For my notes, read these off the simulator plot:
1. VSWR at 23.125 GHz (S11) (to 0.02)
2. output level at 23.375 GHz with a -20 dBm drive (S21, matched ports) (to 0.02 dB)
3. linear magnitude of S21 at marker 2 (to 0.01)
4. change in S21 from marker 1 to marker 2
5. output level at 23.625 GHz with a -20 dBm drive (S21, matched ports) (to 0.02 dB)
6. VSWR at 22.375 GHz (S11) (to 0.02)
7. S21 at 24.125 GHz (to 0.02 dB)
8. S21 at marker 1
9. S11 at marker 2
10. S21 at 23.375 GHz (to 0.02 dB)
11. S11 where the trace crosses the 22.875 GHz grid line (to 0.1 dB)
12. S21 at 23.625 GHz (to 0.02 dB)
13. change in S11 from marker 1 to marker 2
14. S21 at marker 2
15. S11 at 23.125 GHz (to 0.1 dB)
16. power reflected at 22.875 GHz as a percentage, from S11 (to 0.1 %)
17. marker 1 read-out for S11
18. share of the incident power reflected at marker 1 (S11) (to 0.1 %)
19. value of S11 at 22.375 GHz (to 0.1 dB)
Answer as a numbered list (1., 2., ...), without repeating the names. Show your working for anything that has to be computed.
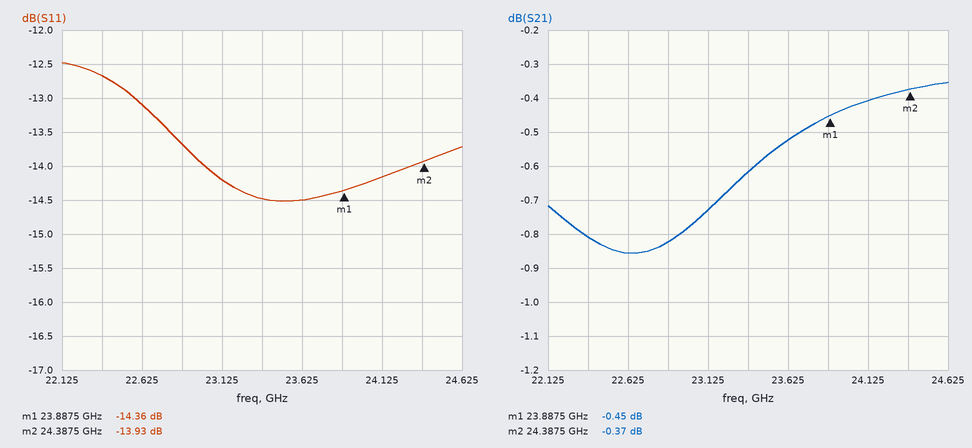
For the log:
1. |Γ| = 10^(-14.2/20) = 0.1950; VSWR = (1 + 0.1950)/(1 − 0.1950) ≈ 1.48
2. -20 dBm + (-0.62 dB) = -20.62 dBm
3. 10^(-0.37/20) ≈ 0.96
4. -0.37 − (-0.45) = 0.08 dB
5. -20 dBm + (-0.52 dB) = -20.52 dBm
6. |Γ| = 10^(-12.7/20) = 0.2317; VSWR = (1 + 0.2317)/(1 − 0.2317) ≈ 1.60
7. -0.40 dB
8. -0.45 dB
9. -13.93 dB
10. -0.62 dB
11. -13.7 dB
12. -0.52 dB
13. -13.93 − (-14.36) = 0.43 dB
14. -0.37 dB
15. -14.2 dB
16. 10^(-13.7/10) ≈ 4.3 %
17. -14.36 dB
18. 10^(-14.36/10) ≈ 3.7 %
19. -12.7 dB
